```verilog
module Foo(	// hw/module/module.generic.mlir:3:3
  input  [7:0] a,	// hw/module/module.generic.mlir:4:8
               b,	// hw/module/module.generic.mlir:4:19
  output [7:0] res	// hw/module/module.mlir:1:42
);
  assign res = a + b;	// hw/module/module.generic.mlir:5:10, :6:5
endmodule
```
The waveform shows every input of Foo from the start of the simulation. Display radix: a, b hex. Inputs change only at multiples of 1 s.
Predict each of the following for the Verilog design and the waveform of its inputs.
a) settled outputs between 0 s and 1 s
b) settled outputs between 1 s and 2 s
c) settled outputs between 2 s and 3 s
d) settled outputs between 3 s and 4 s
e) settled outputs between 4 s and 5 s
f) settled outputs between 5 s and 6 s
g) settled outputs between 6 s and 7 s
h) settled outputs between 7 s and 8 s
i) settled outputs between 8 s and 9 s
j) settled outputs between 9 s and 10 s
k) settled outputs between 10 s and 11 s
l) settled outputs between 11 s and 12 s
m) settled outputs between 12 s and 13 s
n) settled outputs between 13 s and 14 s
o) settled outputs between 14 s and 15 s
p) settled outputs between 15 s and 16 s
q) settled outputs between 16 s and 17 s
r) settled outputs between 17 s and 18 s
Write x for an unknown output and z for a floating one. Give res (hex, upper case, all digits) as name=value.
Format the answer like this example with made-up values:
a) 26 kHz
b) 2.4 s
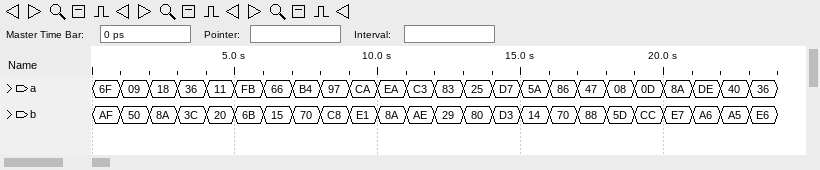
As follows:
a) res=1E
b) res=59
c) res=A2
d) res=72
e) res=31
f) res=66
g) res=7B
h) res=24
i) res=5F
j) res=AB
k) res=74
l) res=71
m) res=AC
n) res=A5
o) res=AA
p) res=6E
q) res=F6
r) res=CF
